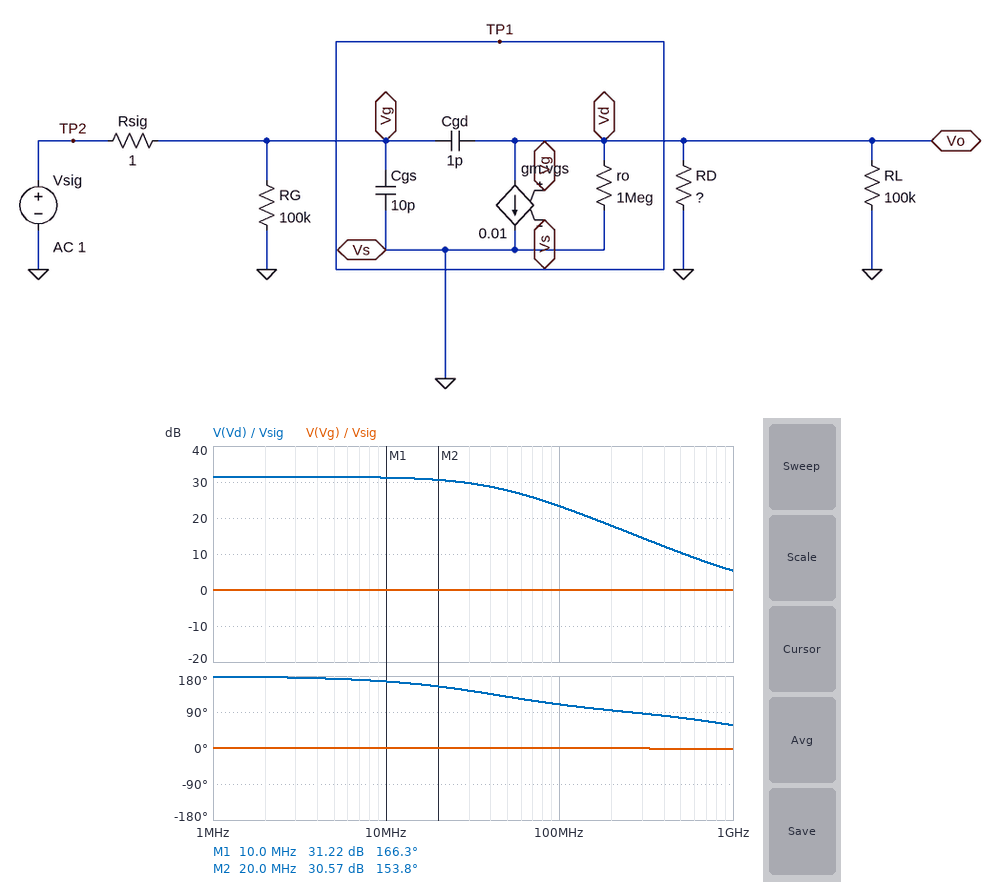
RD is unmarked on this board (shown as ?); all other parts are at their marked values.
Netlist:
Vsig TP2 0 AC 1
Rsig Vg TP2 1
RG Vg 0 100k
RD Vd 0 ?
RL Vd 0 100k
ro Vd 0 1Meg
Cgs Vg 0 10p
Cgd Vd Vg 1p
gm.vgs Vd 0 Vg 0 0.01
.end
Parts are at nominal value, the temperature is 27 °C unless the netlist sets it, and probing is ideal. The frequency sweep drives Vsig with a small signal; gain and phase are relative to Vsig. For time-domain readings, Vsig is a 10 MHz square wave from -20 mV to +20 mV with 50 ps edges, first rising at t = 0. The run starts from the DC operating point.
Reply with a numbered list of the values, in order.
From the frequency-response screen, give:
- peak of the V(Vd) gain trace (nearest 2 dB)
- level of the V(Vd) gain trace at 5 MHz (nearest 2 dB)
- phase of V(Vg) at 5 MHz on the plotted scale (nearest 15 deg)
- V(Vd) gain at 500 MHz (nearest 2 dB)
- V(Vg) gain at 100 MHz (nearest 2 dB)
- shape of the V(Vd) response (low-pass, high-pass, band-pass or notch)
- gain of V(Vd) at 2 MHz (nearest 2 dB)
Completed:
1. 32 dB
2. 32 dB
3. 0 deg
4. 10 dB
5. 0 dB
6. low-pass
7. 32 dB
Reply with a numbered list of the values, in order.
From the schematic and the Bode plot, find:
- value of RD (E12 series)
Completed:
1. 3.9 kΩ
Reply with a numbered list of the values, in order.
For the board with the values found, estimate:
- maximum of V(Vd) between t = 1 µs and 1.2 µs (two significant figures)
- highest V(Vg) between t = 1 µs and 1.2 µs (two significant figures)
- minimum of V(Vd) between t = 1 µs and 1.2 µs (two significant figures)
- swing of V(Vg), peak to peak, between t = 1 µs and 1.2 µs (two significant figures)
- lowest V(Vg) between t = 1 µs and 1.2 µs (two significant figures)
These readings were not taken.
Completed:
1. 770 mV
2. 20 mV
3. -770 mV
4. 40 mV
5. -20 mV
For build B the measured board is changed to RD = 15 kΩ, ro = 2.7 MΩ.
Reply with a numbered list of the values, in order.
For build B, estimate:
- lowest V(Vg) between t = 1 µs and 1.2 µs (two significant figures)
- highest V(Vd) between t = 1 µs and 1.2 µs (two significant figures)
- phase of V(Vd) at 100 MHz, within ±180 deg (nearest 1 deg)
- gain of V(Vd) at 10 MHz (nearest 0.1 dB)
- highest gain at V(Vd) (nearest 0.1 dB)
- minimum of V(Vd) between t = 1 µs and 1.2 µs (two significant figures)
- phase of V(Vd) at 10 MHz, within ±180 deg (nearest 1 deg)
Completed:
1. -20 mV
2. 2.5 V
3. 93 deg
4. 40.0 dB
5. 42.3 dB
6. -2.5 V
7. 140 deg
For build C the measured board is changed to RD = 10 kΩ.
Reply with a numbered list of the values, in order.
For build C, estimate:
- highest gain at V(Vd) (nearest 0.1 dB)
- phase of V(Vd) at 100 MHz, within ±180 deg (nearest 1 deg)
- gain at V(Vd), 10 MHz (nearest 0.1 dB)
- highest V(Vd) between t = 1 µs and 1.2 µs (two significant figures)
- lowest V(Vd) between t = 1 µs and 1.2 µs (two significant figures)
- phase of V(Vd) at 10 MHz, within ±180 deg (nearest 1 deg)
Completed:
1. 39.1 dB
2. 96 deg
3. 37.9 dB
4. 1.8 V
5. -1.8 V
6. 150 deg
